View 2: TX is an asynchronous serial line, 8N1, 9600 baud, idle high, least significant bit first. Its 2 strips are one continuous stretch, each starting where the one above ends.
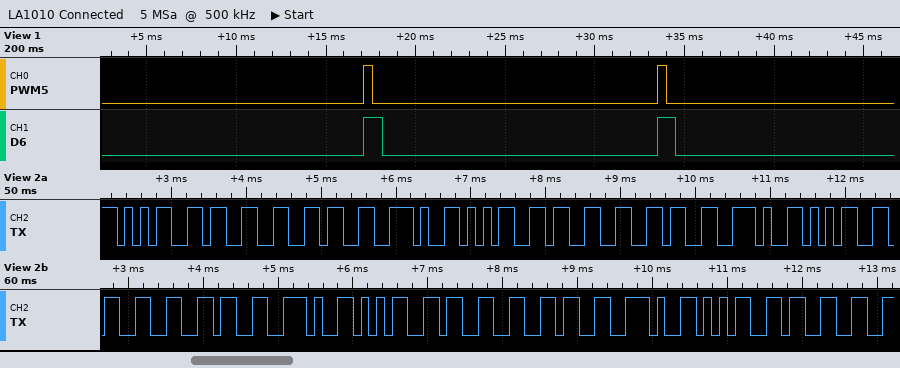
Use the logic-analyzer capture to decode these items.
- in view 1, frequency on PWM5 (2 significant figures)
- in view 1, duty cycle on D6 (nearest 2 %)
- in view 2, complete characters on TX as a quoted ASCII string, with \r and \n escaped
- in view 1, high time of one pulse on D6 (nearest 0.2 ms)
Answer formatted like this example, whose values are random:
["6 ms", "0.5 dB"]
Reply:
["61 Hz", "6 %", "\"536.536.536.536.53\"", "1.0 ms"]
